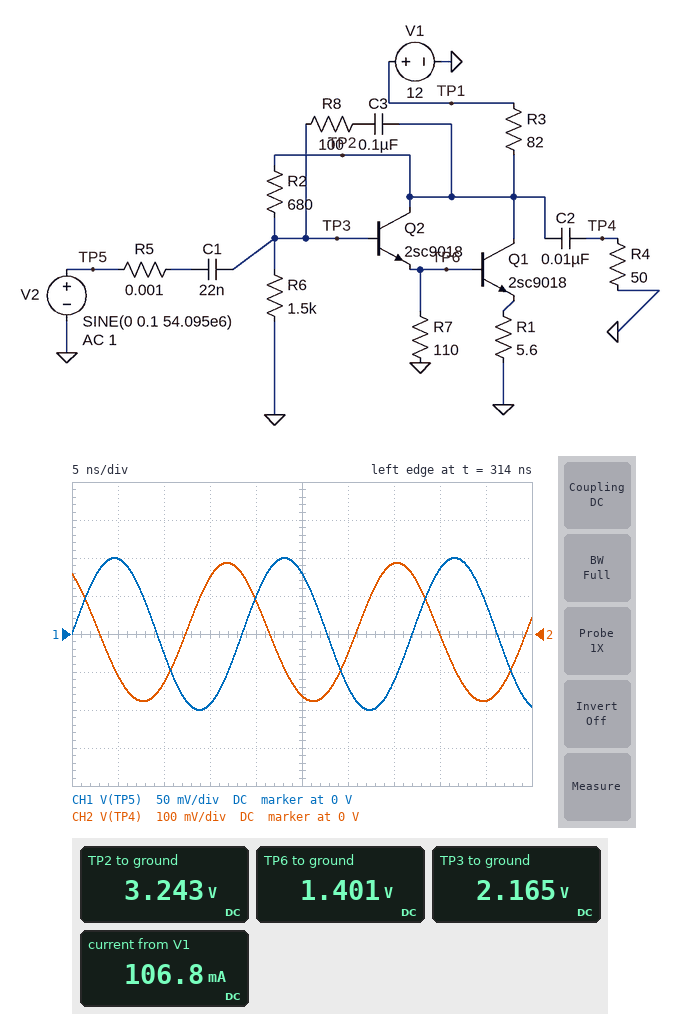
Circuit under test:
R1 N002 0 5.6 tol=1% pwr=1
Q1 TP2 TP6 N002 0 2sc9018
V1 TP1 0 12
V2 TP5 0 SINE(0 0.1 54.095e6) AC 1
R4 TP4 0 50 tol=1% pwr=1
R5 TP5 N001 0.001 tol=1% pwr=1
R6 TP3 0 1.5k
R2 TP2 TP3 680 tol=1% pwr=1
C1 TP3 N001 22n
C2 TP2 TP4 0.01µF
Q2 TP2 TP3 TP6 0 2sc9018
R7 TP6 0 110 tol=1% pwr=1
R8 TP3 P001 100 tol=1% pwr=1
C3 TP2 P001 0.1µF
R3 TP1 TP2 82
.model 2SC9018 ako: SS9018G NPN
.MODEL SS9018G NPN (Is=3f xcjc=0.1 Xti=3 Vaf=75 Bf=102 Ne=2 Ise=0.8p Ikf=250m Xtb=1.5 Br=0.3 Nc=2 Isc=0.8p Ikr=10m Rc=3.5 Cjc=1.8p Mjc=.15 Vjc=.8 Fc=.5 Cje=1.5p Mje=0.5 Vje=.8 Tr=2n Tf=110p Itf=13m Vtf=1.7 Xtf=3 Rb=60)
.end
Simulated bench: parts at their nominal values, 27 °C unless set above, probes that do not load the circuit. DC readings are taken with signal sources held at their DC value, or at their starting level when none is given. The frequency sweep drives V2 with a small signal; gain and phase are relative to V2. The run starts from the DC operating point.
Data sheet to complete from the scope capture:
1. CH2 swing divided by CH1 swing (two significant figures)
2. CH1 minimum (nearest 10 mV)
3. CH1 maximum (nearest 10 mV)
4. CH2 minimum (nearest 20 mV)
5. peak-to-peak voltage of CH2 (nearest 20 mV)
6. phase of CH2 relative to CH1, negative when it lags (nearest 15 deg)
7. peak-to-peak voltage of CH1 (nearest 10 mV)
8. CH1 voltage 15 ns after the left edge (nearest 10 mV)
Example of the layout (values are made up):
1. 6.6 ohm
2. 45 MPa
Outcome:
1. 1.8
2. -100 mV
3. 100 mV
4. -180 mV
5. 360 mV
6. 120 deg
7. 200 mV
8. -90 mV
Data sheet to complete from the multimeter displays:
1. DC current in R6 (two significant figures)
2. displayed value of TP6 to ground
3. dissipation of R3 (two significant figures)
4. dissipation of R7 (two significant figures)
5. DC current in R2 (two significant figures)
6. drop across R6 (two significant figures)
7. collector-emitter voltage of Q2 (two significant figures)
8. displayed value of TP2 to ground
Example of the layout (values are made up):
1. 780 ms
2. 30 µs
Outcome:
1. 1.4 mA
2. 1.401 V
3. 940 mW
4. 18 mW
5. 1.6 mA
6. 2.2 V
7. 1.8 V
8. 3.243 V
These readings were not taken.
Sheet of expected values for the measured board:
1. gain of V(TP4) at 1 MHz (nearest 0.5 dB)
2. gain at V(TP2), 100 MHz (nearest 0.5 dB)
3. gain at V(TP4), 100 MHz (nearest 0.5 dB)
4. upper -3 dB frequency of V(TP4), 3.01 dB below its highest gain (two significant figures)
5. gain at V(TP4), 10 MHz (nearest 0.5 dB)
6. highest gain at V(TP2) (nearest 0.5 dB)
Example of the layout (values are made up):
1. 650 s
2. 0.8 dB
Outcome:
1. 9.5 dB
2. 1.5 dB
3. 1.5 dB
4. 39 MHz
5. 9.5 dB
6. 10.0 dB
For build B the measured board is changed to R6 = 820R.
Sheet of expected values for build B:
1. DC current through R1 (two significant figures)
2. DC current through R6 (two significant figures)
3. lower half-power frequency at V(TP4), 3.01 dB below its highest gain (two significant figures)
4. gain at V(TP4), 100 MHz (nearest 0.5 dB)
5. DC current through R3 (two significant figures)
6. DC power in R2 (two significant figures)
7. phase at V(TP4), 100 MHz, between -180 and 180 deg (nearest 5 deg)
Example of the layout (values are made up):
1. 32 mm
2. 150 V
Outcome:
1. 84 mA
2. 2.6 mA
3. 390 kHz
4. 3.0 dB
5. 98 mA
6. 4.9 mW
7. 110 deg
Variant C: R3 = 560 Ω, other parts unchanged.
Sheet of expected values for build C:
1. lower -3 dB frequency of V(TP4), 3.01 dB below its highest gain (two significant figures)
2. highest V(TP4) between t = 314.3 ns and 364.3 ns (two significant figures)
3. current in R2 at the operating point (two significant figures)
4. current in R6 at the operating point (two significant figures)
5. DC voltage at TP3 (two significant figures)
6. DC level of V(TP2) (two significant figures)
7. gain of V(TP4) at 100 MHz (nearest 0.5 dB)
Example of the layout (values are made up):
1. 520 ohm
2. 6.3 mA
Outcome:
1. 340 kHz
2. 230 mV
3. 1.1 mA
4. 1.0 mA
5. 1.5 V
6. 2.3 V
7. 7.5 dB
